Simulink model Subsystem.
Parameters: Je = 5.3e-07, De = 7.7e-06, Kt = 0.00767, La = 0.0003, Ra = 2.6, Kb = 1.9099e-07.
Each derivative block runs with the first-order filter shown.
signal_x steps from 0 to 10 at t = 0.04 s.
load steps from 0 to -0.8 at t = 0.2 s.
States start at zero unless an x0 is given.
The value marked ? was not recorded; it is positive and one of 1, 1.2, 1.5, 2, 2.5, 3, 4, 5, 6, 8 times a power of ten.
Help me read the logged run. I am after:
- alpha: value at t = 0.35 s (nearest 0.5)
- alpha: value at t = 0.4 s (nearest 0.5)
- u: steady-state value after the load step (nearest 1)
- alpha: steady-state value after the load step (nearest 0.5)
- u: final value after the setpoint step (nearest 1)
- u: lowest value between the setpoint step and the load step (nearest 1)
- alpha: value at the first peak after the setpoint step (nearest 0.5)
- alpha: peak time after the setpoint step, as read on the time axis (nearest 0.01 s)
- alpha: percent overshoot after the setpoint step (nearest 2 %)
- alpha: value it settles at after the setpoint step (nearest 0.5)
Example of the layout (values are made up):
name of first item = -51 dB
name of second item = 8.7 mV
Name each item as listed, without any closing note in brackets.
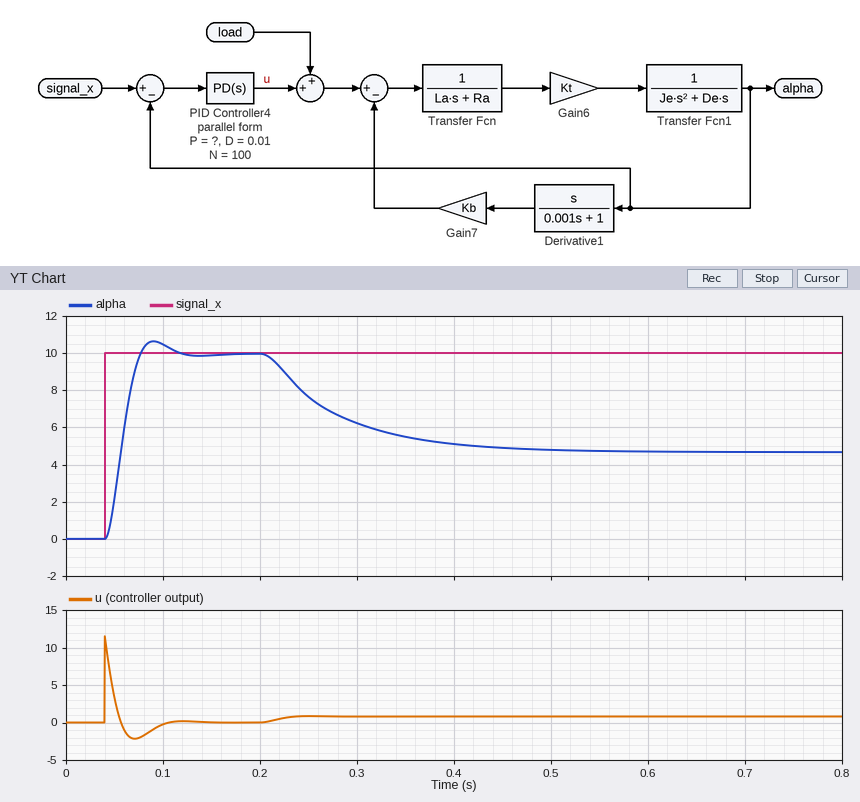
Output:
alpha: value at t = 0.35 s = 5.5
alpha: value at t = 0.4 s = 5.0
u: steady-state value after the load step = 1
alpha: steady-state value after the load step = 4.5
u: final value after the setpoint step = 0
u: lowest value between the setpoint step and the load step = -2
alpha: value at the first peak after the setpoint step = 10.5
alpha: peak time after the setpoint step, as read on the time axis = 0.09 s
alpha: percent overshoot after the setpoint step = 6 %
alpha: value it settles at after the setpoint step = 10.0
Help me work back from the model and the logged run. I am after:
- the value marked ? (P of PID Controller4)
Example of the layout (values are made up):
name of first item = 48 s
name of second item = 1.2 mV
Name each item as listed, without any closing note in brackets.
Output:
the value marked ? = 0.15
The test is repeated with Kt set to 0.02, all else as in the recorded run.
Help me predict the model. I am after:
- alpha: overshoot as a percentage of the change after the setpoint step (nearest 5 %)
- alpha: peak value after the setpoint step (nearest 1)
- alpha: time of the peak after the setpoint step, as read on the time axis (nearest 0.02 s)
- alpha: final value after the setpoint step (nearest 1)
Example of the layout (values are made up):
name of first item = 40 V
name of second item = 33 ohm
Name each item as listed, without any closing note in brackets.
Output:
alpha: overshoot as a percentage of the change after the setpoint step = 25 %
alpha: peak value after the setpoint step = 13
alpha: time of the peak after the setpoint step, as read on the time axis = 0.06 s
alpha: final value after the setpoint step = 10
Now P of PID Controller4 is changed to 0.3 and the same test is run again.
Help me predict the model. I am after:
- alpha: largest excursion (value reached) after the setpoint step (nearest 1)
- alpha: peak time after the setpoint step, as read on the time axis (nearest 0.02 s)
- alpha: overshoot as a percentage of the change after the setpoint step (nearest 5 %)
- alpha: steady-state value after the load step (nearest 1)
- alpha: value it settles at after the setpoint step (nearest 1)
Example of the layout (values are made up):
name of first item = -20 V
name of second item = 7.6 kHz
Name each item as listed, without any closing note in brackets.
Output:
alpha: largest excursion (value reached) after the setpoint step = 12
alpha: peak time after the setpoint step, as read on the time axis = 0.08 s
alpha: overshoot as a percentage of the change after the setpoint step = 20 %
alpha: steady-state value after the load step = 7
alpha: value it settles at after the setpoint step = 10
